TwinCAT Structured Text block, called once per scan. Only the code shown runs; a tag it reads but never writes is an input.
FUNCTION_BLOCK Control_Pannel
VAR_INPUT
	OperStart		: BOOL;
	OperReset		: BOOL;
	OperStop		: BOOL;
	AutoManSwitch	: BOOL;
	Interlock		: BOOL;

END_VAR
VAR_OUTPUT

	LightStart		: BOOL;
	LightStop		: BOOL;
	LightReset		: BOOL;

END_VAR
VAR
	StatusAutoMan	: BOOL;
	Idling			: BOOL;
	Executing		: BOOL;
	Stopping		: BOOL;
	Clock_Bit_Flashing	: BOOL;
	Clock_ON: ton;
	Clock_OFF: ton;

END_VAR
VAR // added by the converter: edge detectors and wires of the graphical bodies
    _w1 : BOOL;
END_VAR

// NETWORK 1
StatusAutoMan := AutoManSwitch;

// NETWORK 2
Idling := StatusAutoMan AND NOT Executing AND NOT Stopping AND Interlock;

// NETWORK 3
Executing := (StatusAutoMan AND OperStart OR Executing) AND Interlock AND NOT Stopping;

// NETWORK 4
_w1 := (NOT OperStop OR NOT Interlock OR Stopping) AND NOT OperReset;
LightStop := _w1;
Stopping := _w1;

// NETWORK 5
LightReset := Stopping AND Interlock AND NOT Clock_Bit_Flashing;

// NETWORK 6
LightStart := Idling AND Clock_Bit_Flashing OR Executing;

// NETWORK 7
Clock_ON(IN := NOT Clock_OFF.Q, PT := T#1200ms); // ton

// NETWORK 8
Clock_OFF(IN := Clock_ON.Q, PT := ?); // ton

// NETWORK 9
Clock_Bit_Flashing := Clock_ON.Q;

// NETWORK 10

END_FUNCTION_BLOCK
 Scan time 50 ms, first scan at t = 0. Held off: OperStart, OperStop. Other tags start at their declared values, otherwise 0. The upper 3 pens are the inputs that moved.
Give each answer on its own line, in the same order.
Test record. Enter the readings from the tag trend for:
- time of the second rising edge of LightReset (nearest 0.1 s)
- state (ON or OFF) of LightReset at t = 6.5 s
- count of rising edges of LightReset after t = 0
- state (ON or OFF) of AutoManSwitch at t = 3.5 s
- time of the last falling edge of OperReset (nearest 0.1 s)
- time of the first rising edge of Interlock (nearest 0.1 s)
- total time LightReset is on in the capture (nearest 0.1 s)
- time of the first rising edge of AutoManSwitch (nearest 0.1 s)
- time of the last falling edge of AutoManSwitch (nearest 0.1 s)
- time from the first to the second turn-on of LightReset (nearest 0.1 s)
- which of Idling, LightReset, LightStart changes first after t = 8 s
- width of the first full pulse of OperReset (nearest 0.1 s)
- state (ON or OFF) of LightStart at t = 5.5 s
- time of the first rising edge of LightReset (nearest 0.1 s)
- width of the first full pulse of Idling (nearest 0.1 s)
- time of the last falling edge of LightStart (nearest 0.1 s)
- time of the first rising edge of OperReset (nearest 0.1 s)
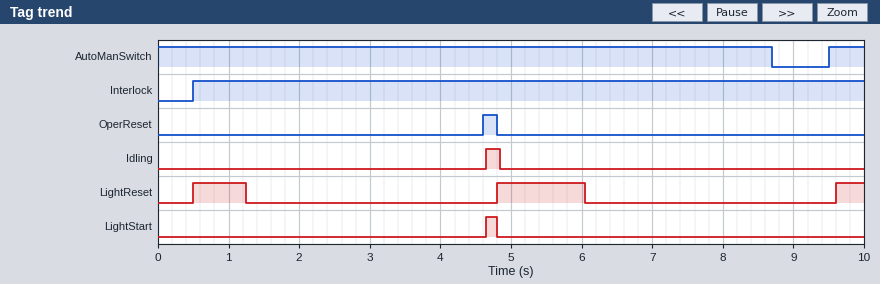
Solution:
4.8 s
OFF
3
ON
4.8 s
0.5 s
2.4 s
9.5 s
8.7 s
4.3 s
LightReset
0.2 s
OFF
0.5 s
0.2 s
4.8 s
4.6 s
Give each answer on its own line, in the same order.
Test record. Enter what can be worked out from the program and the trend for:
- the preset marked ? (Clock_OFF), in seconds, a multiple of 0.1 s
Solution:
3.5 s
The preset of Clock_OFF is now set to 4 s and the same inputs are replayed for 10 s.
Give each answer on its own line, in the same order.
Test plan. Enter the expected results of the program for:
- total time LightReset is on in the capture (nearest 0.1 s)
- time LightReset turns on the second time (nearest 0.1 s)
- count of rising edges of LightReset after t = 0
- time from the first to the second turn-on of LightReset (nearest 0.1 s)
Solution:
2.0 s
5.3 s
2
4.8 s
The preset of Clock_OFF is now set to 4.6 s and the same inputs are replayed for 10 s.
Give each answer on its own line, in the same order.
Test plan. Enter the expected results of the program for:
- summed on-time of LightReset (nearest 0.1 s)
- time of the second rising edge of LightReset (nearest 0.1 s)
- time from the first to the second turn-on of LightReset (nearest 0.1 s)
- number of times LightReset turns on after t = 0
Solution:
2.0 s
5.9 s
5.4 s
2
